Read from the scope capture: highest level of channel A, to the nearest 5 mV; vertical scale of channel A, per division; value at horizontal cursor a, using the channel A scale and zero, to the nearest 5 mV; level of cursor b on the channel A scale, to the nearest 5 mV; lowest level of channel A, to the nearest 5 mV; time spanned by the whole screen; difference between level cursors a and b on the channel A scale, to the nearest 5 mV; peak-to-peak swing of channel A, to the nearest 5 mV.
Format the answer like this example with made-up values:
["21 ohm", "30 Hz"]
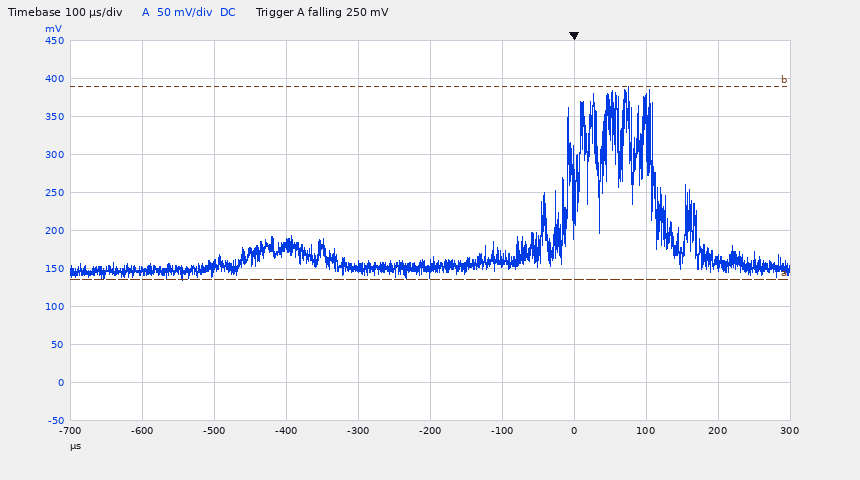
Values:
["390 mV", "50 mV", "135 mV", "390 mV", "135 mV", "1 ms", "255 mV", "255 mV"]
